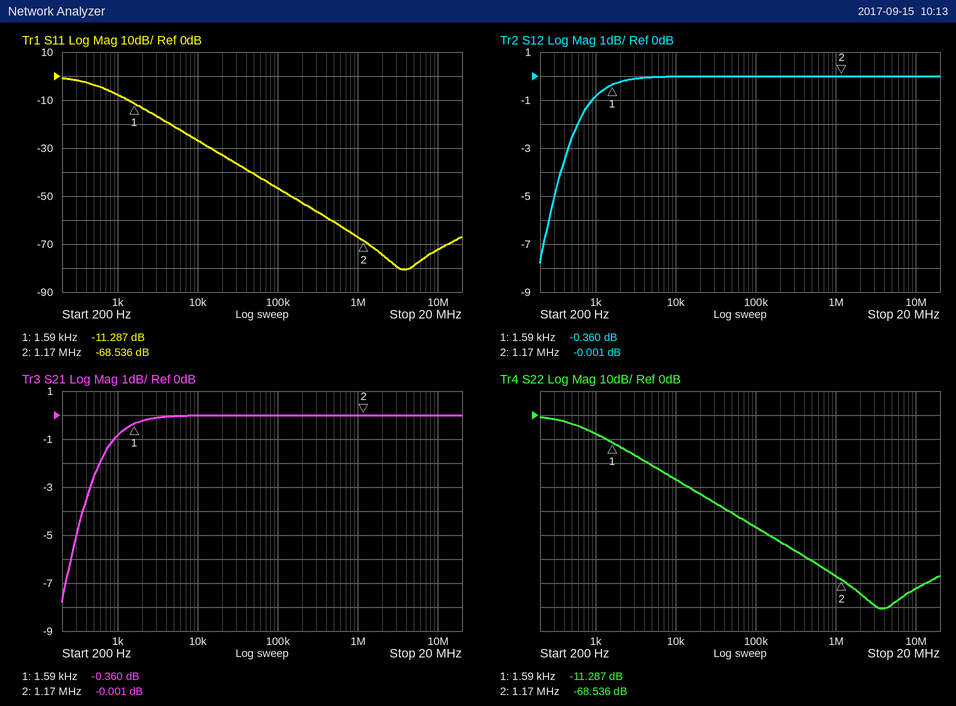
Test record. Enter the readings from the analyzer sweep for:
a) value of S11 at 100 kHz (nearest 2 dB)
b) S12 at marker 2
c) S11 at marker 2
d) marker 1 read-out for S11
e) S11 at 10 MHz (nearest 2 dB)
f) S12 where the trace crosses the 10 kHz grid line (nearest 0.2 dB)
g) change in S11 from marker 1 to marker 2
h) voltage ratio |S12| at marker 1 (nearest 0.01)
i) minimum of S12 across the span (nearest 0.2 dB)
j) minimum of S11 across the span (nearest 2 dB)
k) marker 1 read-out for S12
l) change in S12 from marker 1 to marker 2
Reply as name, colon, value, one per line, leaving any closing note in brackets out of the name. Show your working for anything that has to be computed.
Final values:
value of S11 at 100 kHz: -46 dB
S12 at marker 2: -0.001 dB
S11 at marker 2: -68.536 dB
marker 1 read-out for S11: -11.287 dB
S11 at 10 MHz: -72 dB
S12 where the trace crosses the 10 kHz grid line: 0.0 dB
change in S11 from marker 1 to marker 2: -68.536 − (-11.287) = -57.249 dB
voltage ratio |S12| at marker 1: 10^(-0.36/20) ≈ 0.96
minimum of S12 across the span: -7.8 dB
minimum of S11 across the span: -80 dB
marker 1 read-out for S12: -0.360 dB
change in S12 from marker 1 to marker 2: -0.001 − (-0.36) = 0.359 dB
